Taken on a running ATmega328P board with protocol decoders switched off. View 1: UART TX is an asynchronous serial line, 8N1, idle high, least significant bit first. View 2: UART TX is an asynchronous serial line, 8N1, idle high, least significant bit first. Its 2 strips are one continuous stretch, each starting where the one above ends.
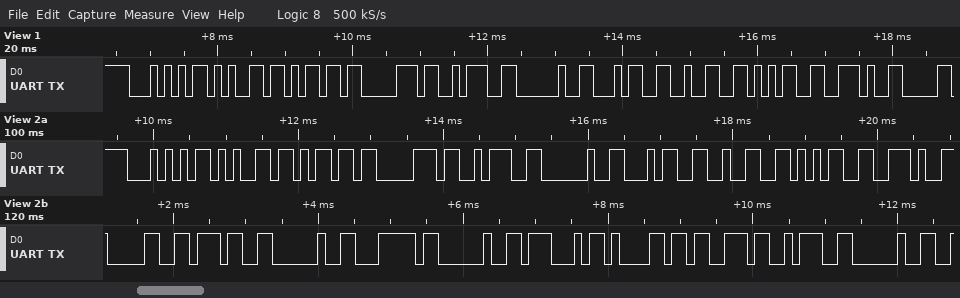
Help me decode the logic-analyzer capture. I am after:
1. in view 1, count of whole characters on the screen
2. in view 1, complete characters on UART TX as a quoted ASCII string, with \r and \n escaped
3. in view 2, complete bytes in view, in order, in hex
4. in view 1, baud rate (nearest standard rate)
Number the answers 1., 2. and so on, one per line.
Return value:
1. 10
2. "Temp: 425."
3. 54 65 6D 70 3A 20 34 32 35 2E 30 37 20 7C 20 47 61 73 3A 20
4. 9600 baud
